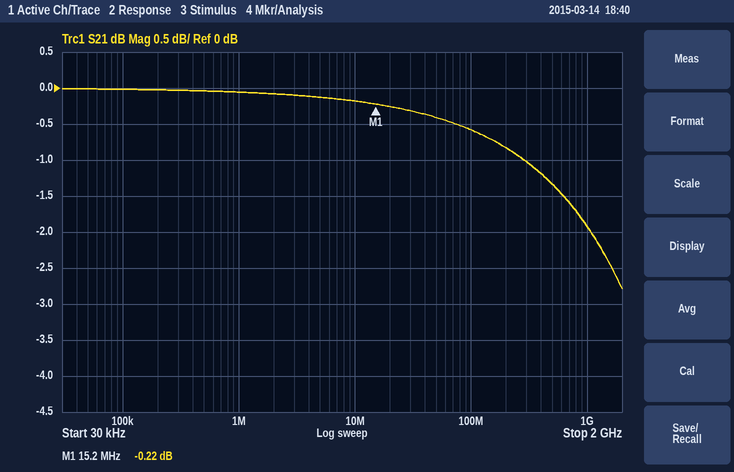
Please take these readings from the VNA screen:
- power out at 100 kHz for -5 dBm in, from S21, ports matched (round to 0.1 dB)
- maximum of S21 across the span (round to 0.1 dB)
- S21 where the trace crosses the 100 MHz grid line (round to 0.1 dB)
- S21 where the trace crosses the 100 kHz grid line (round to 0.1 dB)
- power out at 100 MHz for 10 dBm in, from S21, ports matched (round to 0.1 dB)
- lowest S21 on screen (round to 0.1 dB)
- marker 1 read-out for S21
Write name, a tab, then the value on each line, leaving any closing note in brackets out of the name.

power out at 100 kHz for -5 dBm in, from S21, ports matched	-5.0 dBm
maximum of S21 across the span	0.0 dB
S21 where the trace crosses the 100 MHz grid line	-0.6 dB
S21 where the trace crosses the 100 kHz grid line	0.0 dB
power out at 100 MHz for 10 dBm in, from S21, ports matched	9.4 dBm
lowest S21 on screen	-2.8 dB
marker 1 read-out for S21	-0.22 dB
